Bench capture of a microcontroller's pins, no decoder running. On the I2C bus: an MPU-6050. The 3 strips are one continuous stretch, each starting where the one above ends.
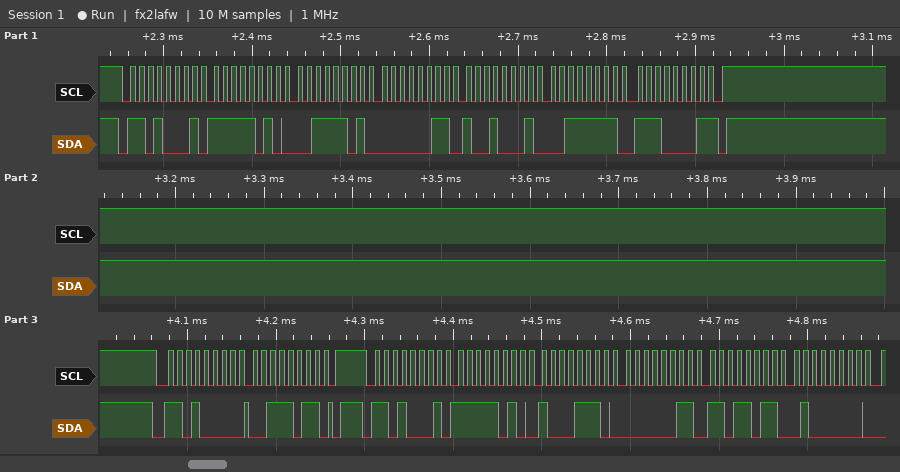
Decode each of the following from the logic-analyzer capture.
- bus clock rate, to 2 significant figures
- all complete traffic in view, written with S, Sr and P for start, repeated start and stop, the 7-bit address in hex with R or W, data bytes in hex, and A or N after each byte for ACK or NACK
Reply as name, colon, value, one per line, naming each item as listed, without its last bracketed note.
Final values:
bus clock rate, to 2 significant figures: 100 kHz
all complete traffic in view, written with S, Sr and P for start, repeated start and stop, the 7-bit address in hex with R or W, data bytes in hex, and A or N after each byte for ACK or NACK: S 68R A FA A 3D A 03 A 91 A 3F A E1 N P S 68W A 3B A P S 68R A FA A 8E A 03 A DB A 40 A
